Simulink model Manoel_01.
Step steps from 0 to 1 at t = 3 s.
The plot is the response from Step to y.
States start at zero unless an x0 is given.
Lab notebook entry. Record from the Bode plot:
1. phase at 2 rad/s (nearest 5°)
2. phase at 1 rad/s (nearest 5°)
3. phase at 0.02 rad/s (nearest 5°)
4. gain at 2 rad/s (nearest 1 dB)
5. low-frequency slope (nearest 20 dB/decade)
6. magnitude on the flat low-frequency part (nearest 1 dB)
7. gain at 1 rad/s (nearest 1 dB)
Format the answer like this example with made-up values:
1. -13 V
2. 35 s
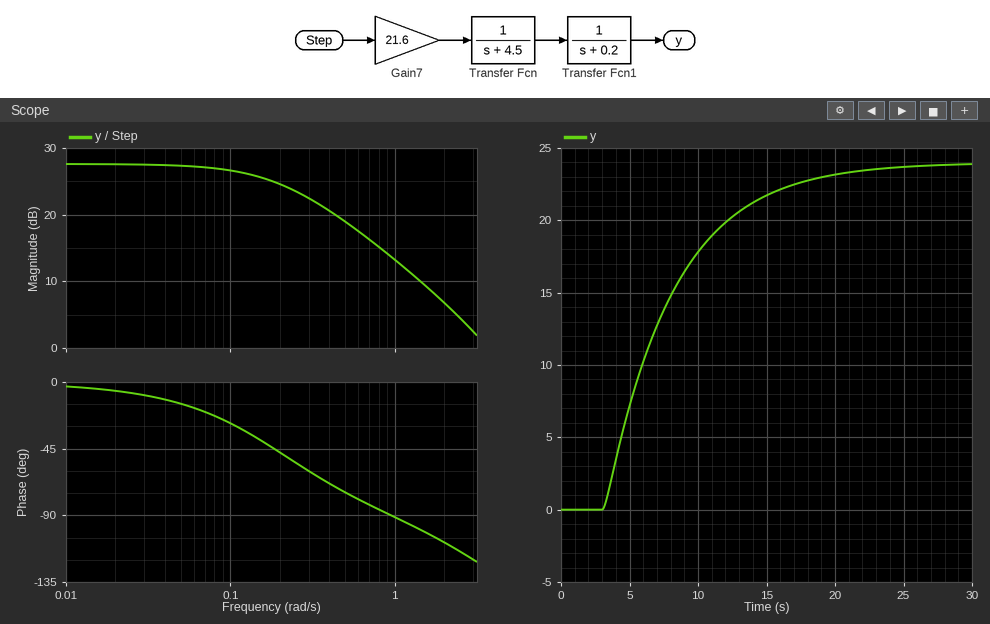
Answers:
1. -110°
2. -90°
3. -5°
4. 7 dB
5. 0 dB/decade
6. 28 dB
7. 13 dB
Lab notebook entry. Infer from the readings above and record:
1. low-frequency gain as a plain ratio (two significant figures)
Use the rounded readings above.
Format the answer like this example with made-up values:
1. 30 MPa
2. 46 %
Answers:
1. 25
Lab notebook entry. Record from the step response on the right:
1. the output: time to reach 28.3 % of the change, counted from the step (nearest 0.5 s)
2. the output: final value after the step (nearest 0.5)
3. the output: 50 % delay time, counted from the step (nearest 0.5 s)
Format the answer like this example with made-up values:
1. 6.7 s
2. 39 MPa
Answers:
1. 2.0 s
2. 24.0
3. 3.5 s
